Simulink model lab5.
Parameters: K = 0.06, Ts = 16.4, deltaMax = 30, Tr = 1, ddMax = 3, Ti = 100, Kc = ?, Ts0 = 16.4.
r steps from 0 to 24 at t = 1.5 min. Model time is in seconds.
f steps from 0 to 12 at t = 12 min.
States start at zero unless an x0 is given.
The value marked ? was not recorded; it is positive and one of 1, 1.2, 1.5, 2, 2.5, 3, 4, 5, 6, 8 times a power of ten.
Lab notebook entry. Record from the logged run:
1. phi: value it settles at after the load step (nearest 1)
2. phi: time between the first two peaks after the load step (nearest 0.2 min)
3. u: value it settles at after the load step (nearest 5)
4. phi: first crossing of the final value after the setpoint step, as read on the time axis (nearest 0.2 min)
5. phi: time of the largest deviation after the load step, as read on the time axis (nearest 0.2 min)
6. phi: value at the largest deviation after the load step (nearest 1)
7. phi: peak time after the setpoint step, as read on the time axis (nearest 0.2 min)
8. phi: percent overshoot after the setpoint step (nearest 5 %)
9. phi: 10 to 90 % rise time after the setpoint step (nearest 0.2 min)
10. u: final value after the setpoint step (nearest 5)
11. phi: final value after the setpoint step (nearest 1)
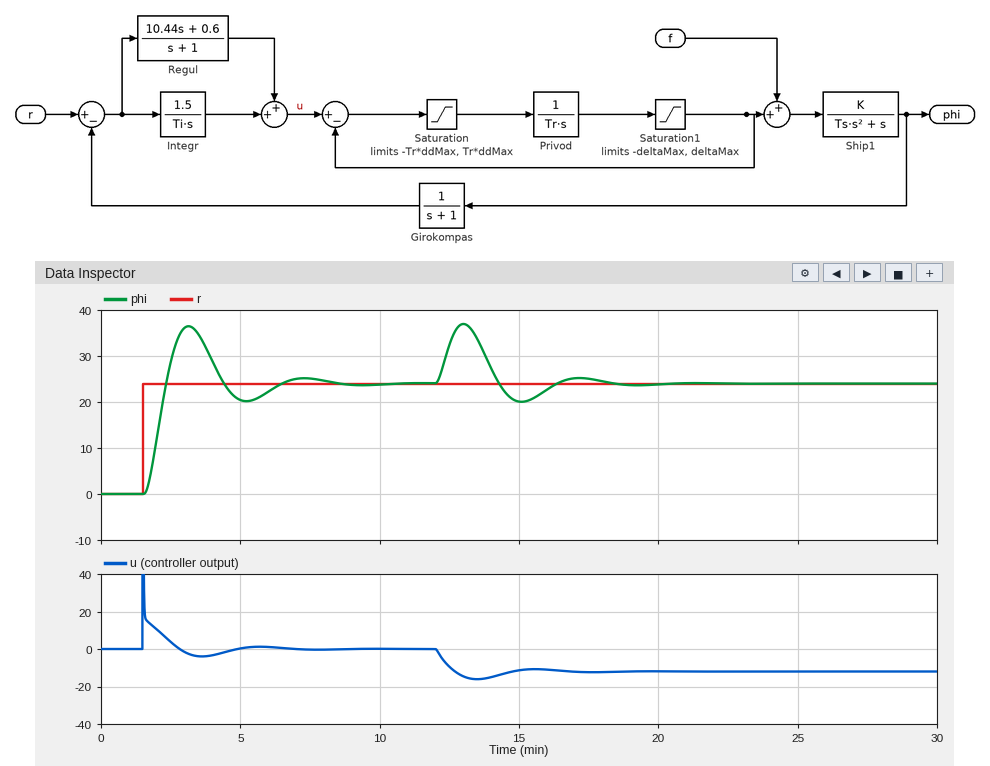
24
4.2 min
-10
2.4 min
13.0 min
37
3.2 min
50 %
0.6 min
0
24
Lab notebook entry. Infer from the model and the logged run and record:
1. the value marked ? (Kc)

0.6
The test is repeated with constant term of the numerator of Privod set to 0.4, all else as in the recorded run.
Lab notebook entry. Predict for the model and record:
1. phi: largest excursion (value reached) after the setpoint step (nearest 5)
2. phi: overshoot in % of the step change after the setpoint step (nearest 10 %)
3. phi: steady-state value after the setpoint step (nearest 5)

40
60 %
25
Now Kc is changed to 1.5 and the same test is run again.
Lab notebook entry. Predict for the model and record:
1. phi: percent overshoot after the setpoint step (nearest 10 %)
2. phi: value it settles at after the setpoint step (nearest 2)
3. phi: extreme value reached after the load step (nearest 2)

20 %
24
30
